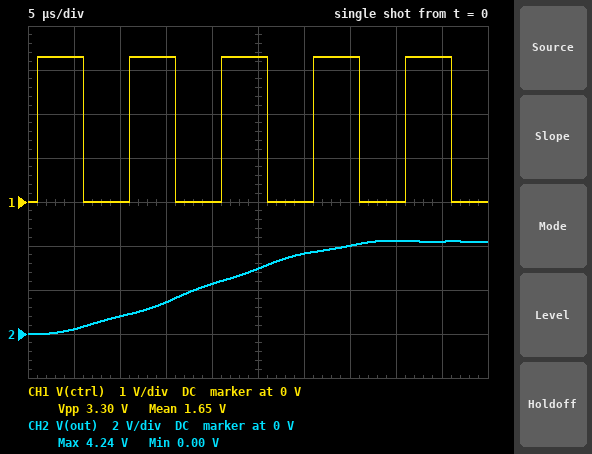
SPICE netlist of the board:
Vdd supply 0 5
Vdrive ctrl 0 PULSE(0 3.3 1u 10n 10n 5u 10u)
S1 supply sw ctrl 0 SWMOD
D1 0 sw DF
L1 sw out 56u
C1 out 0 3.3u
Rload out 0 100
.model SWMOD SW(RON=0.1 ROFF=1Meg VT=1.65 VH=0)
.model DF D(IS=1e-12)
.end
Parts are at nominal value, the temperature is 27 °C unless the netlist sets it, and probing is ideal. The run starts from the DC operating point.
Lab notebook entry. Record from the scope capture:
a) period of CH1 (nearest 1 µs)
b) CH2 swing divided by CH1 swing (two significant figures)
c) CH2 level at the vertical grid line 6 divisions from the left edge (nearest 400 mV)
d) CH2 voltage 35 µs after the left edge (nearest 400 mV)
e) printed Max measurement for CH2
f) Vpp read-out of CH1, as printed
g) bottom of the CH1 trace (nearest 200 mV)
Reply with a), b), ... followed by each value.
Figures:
a) 10 µs
b) 1.3
c) 3.6 V
d) 4.0 V
e) 4.24 V
f) 3.30 V
g) 0 V
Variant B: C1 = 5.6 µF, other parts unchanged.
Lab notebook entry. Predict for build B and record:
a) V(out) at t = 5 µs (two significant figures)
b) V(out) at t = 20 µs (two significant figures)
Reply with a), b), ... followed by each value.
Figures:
a) 130 mV
b) 1.5 V
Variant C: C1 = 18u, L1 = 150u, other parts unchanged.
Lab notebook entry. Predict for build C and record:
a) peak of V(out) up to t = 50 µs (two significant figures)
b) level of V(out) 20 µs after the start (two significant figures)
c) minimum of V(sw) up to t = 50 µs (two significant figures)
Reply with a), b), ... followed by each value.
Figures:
a) 990 mV
b) 190 mV
c) -700 mV
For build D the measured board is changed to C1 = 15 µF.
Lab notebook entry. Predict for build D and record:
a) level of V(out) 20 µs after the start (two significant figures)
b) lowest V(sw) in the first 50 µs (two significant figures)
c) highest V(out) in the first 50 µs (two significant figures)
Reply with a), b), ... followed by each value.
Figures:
a) 600 mV
b) -720 mV
c) 2.6 V
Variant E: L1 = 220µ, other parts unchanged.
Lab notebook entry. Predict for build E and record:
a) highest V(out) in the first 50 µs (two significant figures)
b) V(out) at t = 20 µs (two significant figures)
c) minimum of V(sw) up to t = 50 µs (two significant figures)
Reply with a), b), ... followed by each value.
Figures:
a) 2.8 V
b) 680 mV
c) -680 mV
